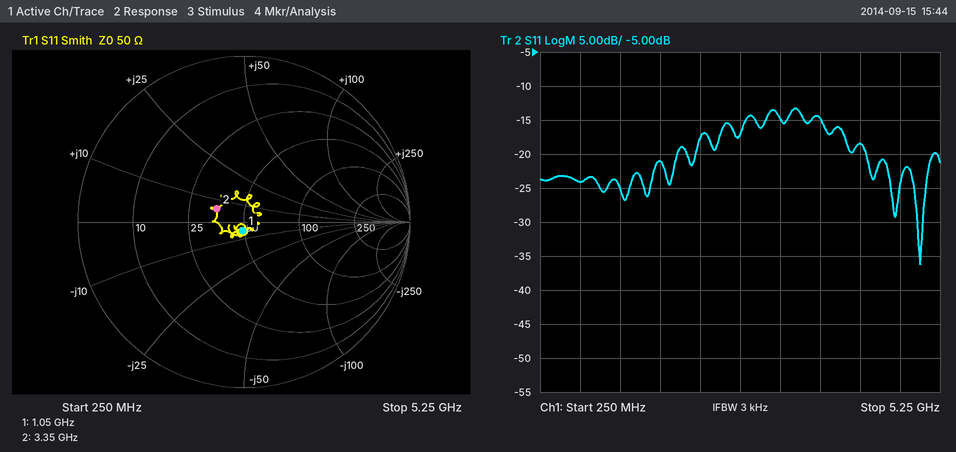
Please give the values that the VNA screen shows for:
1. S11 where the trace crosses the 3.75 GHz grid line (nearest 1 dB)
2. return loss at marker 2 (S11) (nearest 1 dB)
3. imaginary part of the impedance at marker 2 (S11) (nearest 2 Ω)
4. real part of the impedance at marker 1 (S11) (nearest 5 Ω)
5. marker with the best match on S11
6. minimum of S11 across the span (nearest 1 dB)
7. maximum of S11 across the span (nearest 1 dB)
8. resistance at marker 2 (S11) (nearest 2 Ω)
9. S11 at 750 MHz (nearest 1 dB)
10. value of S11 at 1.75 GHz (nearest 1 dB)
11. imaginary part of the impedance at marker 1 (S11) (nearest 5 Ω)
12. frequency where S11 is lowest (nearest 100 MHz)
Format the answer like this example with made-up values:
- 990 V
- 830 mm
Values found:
- -15 dB
- 15 dB
- +6 Ω
- 50 Ω
- marker 1
- -36 dB
- -13 dB
- 36 Ω
- -24 dB
- -21 dB
- -5 Ω
- 5.0 GHz
